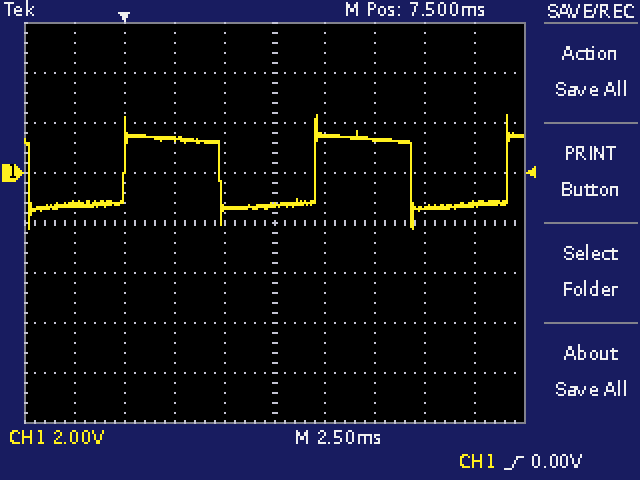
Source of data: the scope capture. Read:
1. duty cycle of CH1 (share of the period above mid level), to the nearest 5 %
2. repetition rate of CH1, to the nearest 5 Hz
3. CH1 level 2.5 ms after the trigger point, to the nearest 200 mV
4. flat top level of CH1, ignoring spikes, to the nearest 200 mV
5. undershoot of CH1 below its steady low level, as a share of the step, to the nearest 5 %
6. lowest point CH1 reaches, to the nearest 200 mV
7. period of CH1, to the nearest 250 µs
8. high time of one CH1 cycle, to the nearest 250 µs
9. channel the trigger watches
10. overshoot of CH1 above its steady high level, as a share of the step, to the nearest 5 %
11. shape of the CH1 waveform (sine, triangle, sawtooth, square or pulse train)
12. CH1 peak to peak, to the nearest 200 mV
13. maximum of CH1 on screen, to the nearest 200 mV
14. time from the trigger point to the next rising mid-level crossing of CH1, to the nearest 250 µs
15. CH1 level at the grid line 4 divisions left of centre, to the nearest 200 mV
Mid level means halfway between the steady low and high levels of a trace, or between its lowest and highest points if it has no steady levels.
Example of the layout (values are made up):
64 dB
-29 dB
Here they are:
50 %
105 Hz
1.4 V
1.4 V
35 %
-2.2 V
9.50 ms
4.75 ms
CH1
35 %
square
4.6 V
2.4 V
9.50 ms
-1.2 V
